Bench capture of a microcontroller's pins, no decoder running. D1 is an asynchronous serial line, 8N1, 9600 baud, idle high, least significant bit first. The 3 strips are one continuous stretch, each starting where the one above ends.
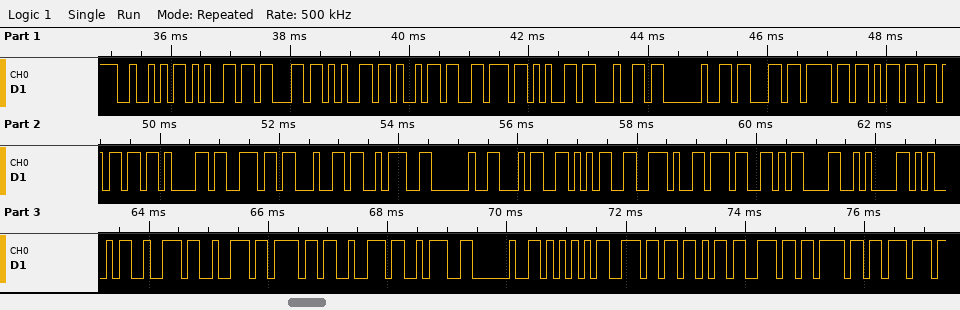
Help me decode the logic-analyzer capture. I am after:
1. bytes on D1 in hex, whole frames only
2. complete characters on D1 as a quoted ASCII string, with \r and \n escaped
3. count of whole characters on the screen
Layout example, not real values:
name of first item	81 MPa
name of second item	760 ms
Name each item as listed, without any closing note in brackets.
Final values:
bytes on D1 in hex, whole frames only	52 65 63 65 69 76 65 64 20 63 6F 6D 6D 61 6E 64 3A 20 34 35 2E 37 0D 0A 45 72 72 6F 72 3A 20 55 6E 6B 6E 6F 77
complete characters on D1 as a quoted ASCII string, with \r and \n escaped	"Received command: 45.7\r\nError: Unknow"
count of whole characters on the screen	37
